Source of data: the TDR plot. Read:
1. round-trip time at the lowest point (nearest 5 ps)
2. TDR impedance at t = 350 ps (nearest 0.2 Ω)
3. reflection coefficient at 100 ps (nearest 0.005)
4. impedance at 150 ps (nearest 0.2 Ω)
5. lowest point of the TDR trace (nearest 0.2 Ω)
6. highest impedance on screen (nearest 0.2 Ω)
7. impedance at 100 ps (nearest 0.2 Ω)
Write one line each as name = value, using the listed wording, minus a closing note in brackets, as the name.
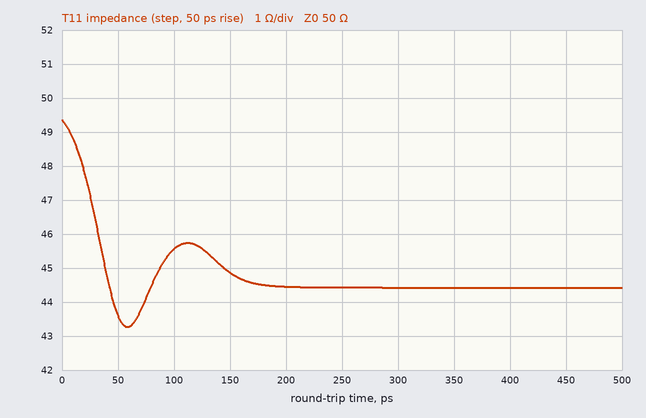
round-trip time at the lowest point = 60 ps
TDR impedance at t = 350 ps = 44.4 Ω
reflection coefficient at 100 ps = -0.045
impedance at 150 ps = 44.8 Ω
lowest point of the TDR trace = 43.2 Ω
highest impedance on screen = 49.4 Ω
impedance at 100 ps = 45.6 Ω
